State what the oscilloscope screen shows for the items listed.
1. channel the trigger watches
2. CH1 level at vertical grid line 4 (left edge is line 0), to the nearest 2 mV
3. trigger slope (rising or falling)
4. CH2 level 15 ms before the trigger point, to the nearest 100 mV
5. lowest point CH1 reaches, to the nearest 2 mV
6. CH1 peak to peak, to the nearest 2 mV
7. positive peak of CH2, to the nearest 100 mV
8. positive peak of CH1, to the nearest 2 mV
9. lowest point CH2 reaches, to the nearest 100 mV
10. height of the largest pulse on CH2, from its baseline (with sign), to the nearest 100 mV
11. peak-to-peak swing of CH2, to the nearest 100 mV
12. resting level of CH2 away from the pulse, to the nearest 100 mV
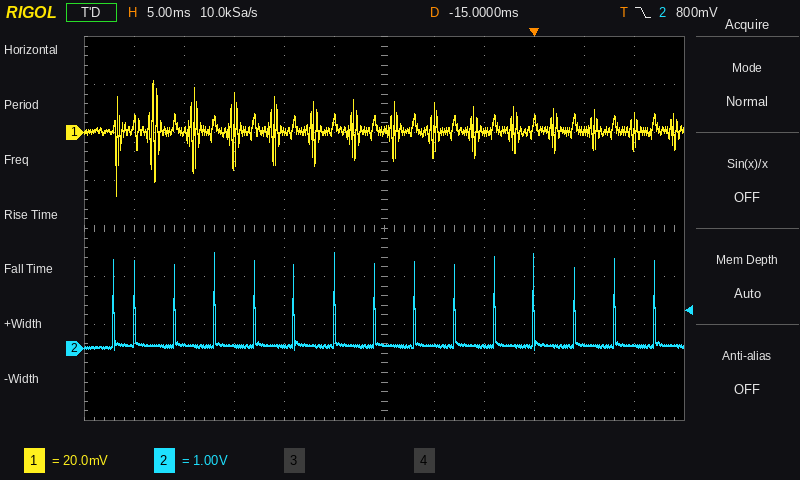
CH2
0 mV
falling
100 mV
-26 mV
48 mV
2.0 V
22 mV
0.0 V
+1.9 V
2.0 V
100 mV
